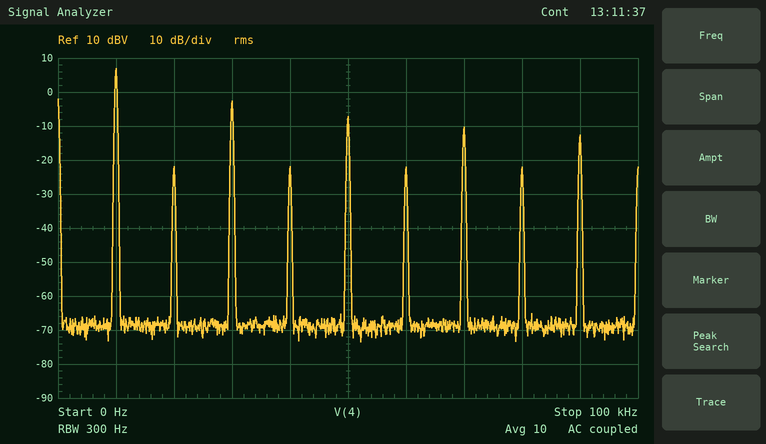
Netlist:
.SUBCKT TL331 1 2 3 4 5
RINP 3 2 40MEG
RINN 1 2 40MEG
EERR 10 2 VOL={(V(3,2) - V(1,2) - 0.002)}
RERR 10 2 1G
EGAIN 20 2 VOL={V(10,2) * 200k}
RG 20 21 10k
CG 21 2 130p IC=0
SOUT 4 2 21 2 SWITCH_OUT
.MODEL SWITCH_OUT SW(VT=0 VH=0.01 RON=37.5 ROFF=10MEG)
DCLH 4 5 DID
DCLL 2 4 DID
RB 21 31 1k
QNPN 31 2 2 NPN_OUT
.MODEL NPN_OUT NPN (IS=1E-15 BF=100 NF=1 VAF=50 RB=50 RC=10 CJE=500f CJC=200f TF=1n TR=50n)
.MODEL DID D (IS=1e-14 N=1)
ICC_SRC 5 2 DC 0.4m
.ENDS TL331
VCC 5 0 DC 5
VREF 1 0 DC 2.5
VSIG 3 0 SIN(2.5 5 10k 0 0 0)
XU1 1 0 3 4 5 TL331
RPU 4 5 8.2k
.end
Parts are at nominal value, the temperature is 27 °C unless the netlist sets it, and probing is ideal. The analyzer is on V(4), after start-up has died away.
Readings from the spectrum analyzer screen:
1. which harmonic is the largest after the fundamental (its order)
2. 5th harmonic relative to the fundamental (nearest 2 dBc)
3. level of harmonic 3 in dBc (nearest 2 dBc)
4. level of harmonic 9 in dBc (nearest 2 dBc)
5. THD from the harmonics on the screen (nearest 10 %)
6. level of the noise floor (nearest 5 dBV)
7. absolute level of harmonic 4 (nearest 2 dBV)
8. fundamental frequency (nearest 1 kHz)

3
-14 dBc
-10 dBc
-20 dBc
40 %
-70 dBV
-22 dBV
10 kHz
